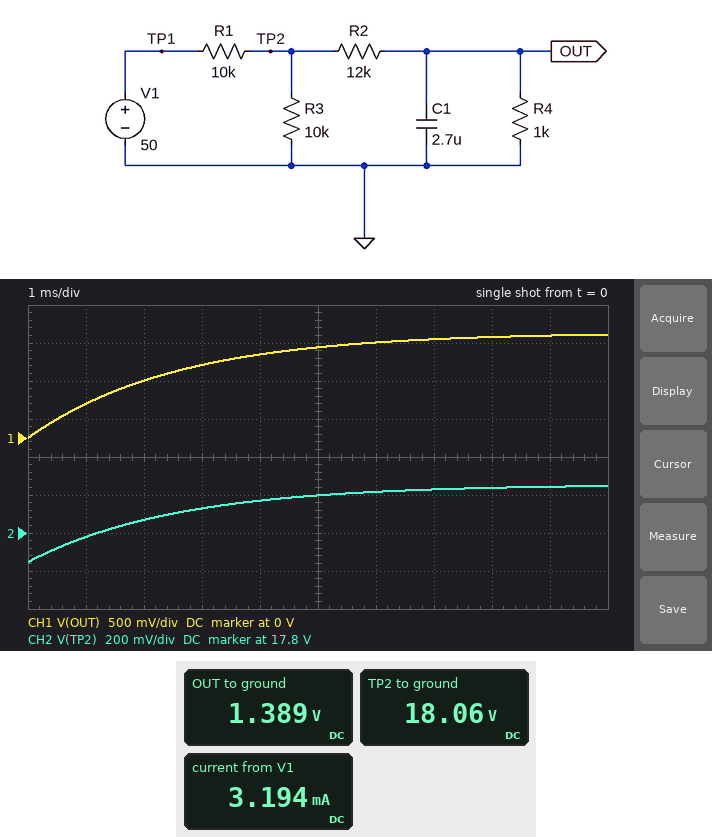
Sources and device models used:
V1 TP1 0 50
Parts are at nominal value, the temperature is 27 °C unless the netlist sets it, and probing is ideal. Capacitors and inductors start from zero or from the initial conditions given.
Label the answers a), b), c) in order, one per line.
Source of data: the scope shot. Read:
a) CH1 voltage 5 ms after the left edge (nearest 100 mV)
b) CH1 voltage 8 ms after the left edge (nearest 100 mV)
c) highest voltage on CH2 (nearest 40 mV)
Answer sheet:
a) 1.2 V
b) 1.3 V
c) 18.04 V
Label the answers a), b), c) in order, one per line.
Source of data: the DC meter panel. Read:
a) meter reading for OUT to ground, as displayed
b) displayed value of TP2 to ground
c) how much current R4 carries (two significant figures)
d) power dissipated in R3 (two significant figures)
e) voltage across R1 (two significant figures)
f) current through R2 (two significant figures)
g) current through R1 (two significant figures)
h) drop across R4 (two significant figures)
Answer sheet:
a) 1.389 V
b) 18.06 V
c) 1.4 mA
d) 33 mW
e) 32 V
f) 1.4 mA
g) 3.2 mA
h) 1.4 V
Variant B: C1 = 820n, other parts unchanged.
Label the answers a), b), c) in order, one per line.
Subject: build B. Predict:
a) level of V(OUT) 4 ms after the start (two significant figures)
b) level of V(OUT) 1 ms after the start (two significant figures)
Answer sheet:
a) 1.4 V
b) 1.0 V
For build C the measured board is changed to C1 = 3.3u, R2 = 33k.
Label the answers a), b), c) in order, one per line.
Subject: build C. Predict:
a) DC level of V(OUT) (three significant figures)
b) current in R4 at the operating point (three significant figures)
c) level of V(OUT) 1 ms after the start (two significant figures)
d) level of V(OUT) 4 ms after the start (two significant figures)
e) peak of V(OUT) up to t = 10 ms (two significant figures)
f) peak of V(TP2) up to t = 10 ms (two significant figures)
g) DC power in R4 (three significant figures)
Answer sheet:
a) 641 mV
b) 641 µA
c) 170 mV
d) 460 mV
e) 610 mV
f) 22 V
g) 411 µW
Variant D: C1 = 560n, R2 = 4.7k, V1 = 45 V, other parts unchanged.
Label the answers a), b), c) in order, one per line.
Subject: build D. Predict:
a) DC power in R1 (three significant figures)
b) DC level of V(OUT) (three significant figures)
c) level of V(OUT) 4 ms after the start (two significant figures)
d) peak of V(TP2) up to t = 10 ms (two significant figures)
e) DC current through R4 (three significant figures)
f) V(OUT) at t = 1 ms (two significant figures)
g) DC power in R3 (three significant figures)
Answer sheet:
a) 109 mW
b) 2.10 V
c) 2.1 V
d) 12 V
e) 2.10 mA
f) 1.8 V
g) 14.4 mW
